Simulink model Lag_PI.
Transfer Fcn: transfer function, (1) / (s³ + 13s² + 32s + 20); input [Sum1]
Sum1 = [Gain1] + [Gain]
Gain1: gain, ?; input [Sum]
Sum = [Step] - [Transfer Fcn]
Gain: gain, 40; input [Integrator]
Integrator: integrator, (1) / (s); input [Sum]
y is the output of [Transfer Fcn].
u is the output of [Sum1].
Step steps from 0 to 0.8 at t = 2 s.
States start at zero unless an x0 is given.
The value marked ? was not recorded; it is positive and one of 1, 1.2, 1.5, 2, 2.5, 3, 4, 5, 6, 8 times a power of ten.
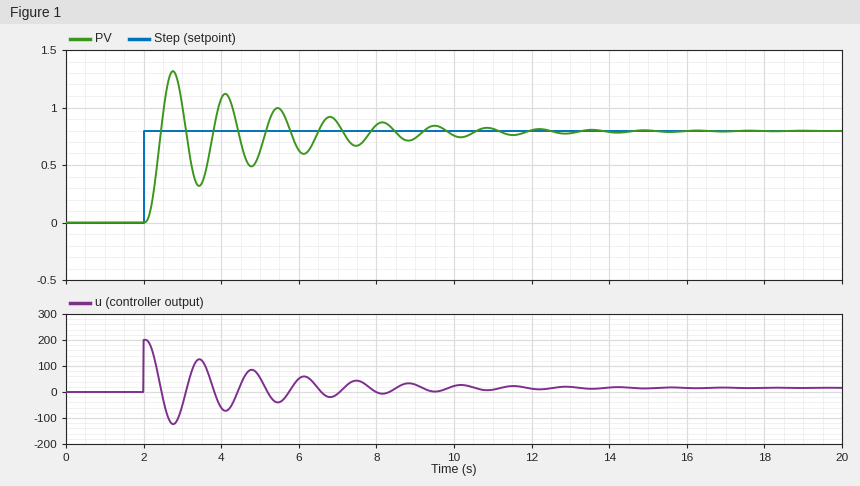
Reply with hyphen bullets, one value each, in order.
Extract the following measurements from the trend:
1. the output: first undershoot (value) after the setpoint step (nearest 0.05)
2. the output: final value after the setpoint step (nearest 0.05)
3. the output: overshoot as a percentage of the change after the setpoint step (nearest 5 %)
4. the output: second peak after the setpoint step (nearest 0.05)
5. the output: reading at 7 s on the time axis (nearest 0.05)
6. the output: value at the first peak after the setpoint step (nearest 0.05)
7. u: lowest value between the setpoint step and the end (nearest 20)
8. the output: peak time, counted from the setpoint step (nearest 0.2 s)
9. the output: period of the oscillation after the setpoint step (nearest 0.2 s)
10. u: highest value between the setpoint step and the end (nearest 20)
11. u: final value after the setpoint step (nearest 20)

- 0.30
- 0.80
- 65 %
- 1.10
- 0.85
- 1.30
- -120
- 0.8 s
- 1.4 s
- 200
- 20
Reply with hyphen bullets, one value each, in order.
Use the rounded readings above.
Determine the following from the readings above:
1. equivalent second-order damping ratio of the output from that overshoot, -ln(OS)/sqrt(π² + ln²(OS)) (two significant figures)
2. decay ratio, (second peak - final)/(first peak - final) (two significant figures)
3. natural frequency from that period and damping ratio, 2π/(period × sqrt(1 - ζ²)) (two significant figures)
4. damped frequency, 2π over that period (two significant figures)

- 0.14
- 0.60
- 4.5 rad/s
- 4.5 rad/s
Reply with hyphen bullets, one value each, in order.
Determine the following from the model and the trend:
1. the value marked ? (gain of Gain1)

- 250
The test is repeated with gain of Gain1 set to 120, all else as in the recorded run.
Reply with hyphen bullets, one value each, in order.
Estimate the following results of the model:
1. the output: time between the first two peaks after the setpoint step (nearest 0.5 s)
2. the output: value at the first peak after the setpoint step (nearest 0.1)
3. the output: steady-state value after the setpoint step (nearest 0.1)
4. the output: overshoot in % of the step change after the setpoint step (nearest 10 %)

- 2.0 s
- 1.1
- 0.8
- 40 %
